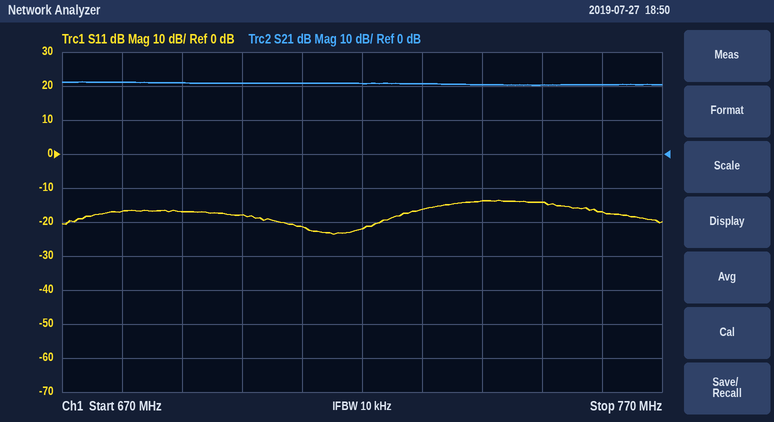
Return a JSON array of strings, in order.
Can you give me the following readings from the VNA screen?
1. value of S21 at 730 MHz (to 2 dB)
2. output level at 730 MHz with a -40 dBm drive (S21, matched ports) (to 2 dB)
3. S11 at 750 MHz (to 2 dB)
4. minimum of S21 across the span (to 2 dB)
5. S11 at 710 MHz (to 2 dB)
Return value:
["20 dB", "-20 dBm", "-14 dB", "20 dB", "-22 dB"]
